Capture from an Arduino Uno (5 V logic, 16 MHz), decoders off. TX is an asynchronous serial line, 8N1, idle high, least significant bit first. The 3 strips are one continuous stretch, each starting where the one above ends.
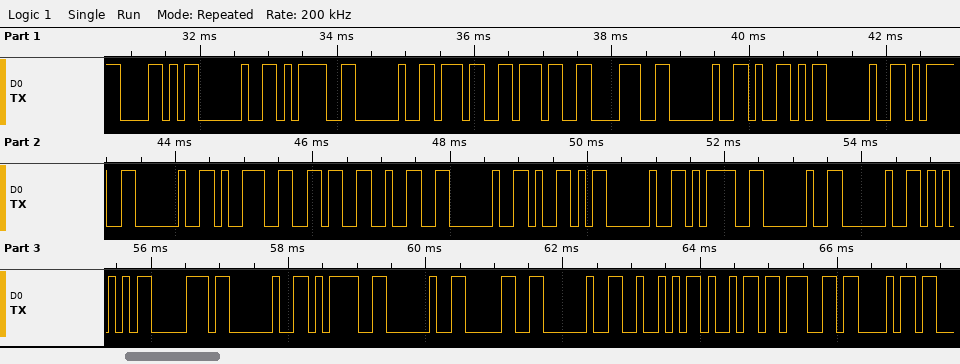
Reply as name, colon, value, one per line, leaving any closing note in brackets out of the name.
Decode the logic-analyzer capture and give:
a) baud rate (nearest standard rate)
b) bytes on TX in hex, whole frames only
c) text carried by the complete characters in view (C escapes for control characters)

baud rate: 9600 baud
bytes on TX in hex, whole frames only: 58 20 3D 20 37 37 38 20 59 20 3D 20 39 36 32 20 59 20 3D 20 20 55 70 20 3D 20 30 20 52 69 67 68
text carried by the complete characters in view: "X = 778 Y = 962 Y =  Up = 0 Righ"
